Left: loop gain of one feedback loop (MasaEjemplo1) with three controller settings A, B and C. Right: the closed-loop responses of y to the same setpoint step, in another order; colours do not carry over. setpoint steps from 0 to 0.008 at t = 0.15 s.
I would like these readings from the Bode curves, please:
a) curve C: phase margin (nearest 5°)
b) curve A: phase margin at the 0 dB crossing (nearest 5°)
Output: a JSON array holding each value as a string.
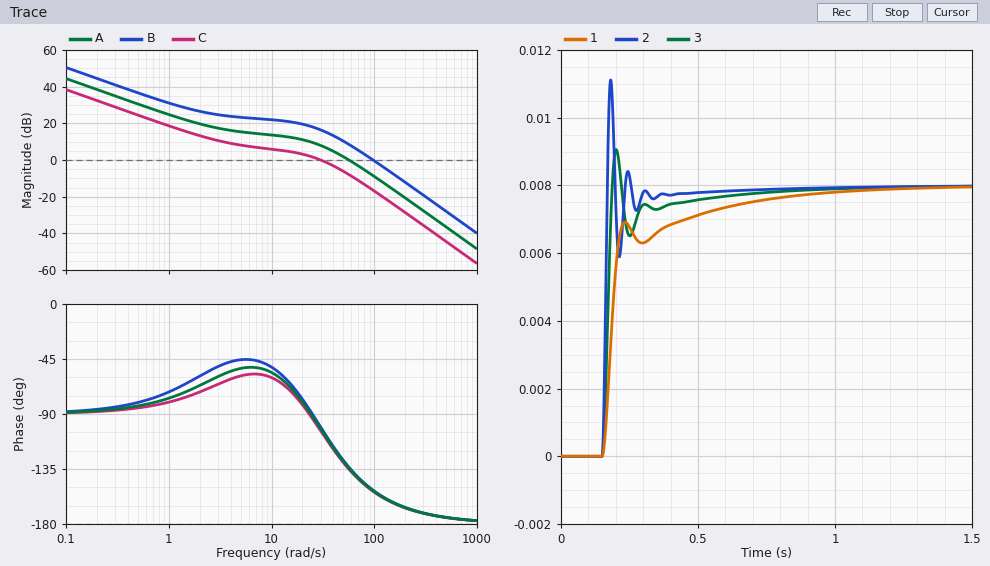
["75°", "45°"]
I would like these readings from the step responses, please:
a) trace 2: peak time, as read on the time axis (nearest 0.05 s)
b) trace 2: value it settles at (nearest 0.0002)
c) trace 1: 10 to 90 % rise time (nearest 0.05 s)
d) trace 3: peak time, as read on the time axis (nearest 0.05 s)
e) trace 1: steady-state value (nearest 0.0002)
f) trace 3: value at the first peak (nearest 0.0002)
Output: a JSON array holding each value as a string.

["0.20 s", "0.0080", "0.35 s", "0.20 s", "0.0080", "0.0090"]
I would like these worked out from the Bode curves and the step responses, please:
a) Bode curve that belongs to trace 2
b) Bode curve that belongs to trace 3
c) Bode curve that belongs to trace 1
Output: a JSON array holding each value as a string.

["B", "A", "C"]
